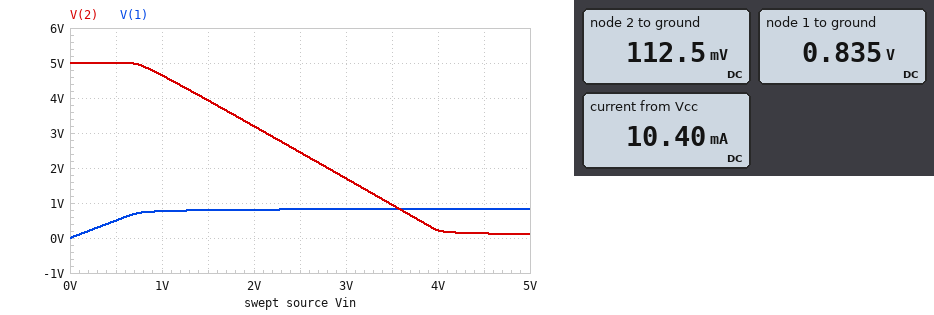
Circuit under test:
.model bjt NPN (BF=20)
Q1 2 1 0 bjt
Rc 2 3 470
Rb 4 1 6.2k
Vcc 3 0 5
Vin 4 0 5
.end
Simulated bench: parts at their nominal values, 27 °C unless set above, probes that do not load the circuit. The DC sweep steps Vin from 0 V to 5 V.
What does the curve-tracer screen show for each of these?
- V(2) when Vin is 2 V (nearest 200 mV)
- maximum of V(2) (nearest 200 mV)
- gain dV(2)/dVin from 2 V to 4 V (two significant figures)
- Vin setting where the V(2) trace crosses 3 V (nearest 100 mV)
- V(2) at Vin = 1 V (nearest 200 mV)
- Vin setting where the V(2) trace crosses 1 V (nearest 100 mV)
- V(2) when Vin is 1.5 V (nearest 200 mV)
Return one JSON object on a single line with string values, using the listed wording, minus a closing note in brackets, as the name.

{"V(2) when Vin is 2 V": "3.2 V", "maximum of V(2)": "5.0 V", "gain dV(2)/dVin from 2 V to 4 V": "-1.5 V/V", "Vin setting where the V(2) trace crosses 3 V": "2.1 V", "V(2) at Vin = 1 V": "4.6 V", "Vin setting where the V(2) trace crosses 1 V": "3.5 V", "V(2) when Vin is 1.5 V": "4.0 V"}
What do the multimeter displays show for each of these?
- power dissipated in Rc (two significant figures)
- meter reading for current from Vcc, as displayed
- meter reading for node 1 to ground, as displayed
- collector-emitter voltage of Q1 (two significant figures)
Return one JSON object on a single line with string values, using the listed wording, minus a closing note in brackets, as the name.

{"power dissipated in Rc": "51 mW", "meter reading for current from Vcc, as displayed": "10.40 mA", "meter reading for node 1 to ground, as displayed": "0.835 V", "collector-emitter voltage of Q1": "110 mV"}
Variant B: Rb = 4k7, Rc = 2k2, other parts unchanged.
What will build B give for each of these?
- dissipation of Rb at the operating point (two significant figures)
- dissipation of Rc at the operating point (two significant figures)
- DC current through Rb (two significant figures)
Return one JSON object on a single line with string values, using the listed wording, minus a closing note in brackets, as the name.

{"dissipation of Rb at the operating point": "3.7 mW", "dissipation of Rc at the operating point": "11 mW", "DC current through Rb": "890 µA"}
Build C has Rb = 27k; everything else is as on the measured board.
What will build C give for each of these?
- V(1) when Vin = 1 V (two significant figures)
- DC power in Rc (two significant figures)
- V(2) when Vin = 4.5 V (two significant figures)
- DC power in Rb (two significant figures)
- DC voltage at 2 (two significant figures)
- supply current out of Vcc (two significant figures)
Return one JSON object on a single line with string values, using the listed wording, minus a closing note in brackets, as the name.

{"V(1) when Vin = 1 V": "730 mV", "DC power in Rc": "4.5 mW", "V(2) when Vin = 4.5 V": "3.7 V", "DC power in Rb": "650 µW", "DC voltage at 2": "3.5 V", "supply current out of Vcc": "3.1 mA"}
